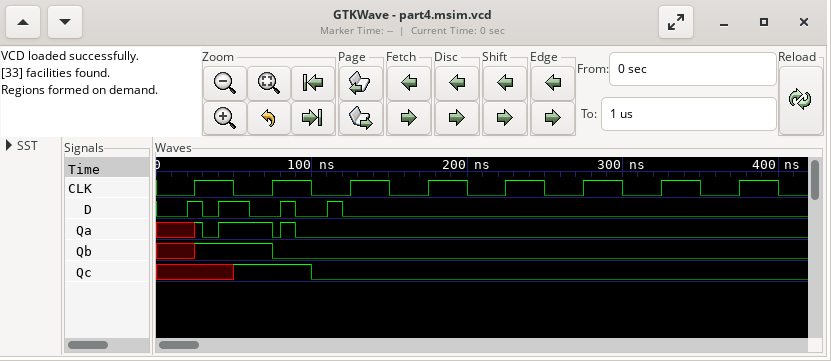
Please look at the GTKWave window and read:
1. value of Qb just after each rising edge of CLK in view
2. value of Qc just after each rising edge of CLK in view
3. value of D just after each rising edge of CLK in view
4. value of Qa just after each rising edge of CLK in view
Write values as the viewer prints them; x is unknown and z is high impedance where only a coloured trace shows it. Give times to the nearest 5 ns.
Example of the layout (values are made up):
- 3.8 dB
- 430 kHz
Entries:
- 1 0 0 0 0 0 0 0
- x 1 0 0 0 0 0 0
- 1 0 0 0 0 0 0 0
- 1 0 0 0 0 0 0 0
